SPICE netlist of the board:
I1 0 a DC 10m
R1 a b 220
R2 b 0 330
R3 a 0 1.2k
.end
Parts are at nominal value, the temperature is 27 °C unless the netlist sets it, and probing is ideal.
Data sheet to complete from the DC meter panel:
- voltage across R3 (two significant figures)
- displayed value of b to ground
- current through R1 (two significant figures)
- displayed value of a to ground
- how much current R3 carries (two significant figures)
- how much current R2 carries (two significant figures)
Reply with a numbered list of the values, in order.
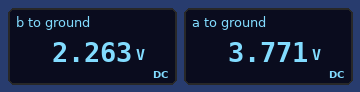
1. 3.8 V
2. 2.263 V
3. 6.9 mA
4. 3.771 V
5. 3.1 mA
6. 6.9 mA
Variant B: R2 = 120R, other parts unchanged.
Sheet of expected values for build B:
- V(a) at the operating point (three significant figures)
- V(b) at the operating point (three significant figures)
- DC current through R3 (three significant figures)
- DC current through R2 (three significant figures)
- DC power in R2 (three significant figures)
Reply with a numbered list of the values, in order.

1. 2.65 V
2. 935 mV
3. 2.21 mA
4. 7.79 mA
5. 7.29 mW
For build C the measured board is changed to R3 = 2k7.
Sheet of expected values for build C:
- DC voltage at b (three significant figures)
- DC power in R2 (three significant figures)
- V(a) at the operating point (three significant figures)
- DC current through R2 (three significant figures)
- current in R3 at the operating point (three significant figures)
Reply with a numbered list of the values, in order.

1. 2.74 V
2. 22.8 mW
3. 4.57 V
4. 8.31 mA
5. 1.69 mA
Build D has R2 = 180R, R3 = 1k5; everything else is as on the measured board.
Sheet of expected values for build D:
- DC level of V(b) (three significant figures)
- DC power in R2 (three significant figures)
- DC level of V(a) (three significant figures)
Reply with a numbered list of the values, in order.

1. 1.42 V
2. 11.2 mW
3. 3.16 V
